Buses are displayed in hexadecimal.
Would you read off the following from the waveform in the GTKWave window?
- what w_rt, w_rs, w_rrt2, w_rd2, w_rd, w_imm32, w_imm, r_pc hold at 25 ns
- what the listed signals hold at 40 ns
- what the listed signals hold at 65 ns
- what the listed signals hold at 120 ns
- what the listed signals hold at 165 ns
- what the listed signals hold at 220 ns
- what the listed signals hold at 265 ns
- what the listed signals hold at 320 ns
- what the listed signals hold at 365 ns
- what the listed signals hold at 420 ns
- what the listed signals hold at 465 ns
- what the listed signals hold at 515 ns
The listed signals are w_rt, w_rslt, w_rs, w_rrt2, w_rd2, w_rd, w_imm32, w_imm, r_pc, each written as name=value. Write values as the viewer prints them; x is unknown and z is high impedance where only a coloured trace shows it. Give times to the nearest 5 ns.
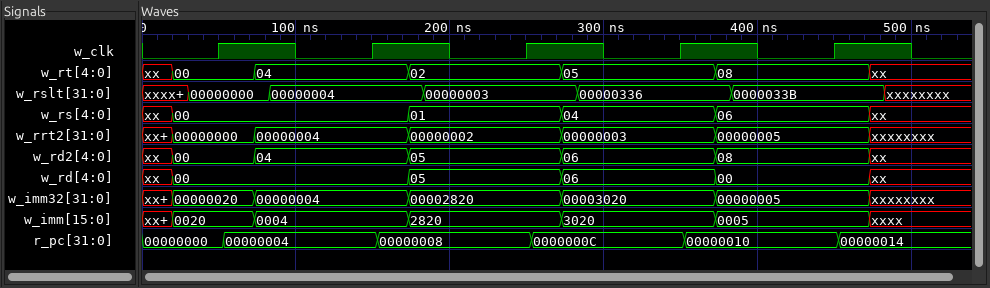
w_rt=00, w_rs=00, w_rrt2=00000000, w_rd2=00, w_rd=00, w_imm32=00000020, w_imm=0020, r_pc=00000000
w_rt=00, w_rslt=00000000, w_rs=00, w_rrt2=00000000, w_rd2=00, w_rd=00, w_imm32=00000020, w_imm=0020, r_pc=00000000
w_rt=00, w_rslt=00000000, w_rs=00, w_rrt2=00000000, w_rd2=00, w_rd=00, w_imm32=00000020, w_imm=0020, r_pc=00000004
w_rt=04, w_rslt=00000004, w_rs=00, w_rrt2=00000004, w_rd2=04, w_rd=00, w_imm32=00000004, w_imm=0004, r_pc=00000004
w_rt=04, w_rslt=00000004, w_rs=00, w_rrt2=00000004, w_rd2=04, w_rd=00, w_imm32=00000004, w_imm=0004, r_pc=00000008
w_rt=02, w_rslt=00000003, w_rs=01, w_rrt2=00000002, w_rd2=05, w_rd=05, w_imm32=00002820, w_imm=2820, r_pc=00000008
w_rt=02, w_rslt=00000003, w_rs=01, w_rrt2=00000002, w_rd2=05, w_rd=05, w_imm32=00002820, w_imm=2820, r_pc=0000000C
w_rt=05, w_rslt=00000336, w_rs=04, w_rrt2=00000003, w_rd2=06, w_rd=06, w_imm32=00003020, w_imm=3020, r_pc=0000000C
w_rt=05, w_rslt=00000336, w_rs=04, w_rrt2=00000003, w_rd2=06, w_rd=06, w_imm32=00003020, w_imm=3020, r_pc=00000010
w_rt=08, w_rslt=0000033B, w_rs=06, w_rrt2=00000005, w_rd2=08, w_rd=00, w_imm32=00000005, w_imm=0005, r_pc=00000010
w_rt=08, w_rslt=0000033B, w_rs=06, w_rrt2=00000005, w_rd2=08, w_rd=00, w_imm32=00000005, w_imm=0005, r_pc=00000014
w_rt=xx, w_rslt=xxxxxxxx, w_rs=xx, w_rrt2=xxxxxxxx, w_rd2=xx, w_rd=xx, w_imm32=xxxxxxxx, w_imm=xxxx, r_pc=00000014
